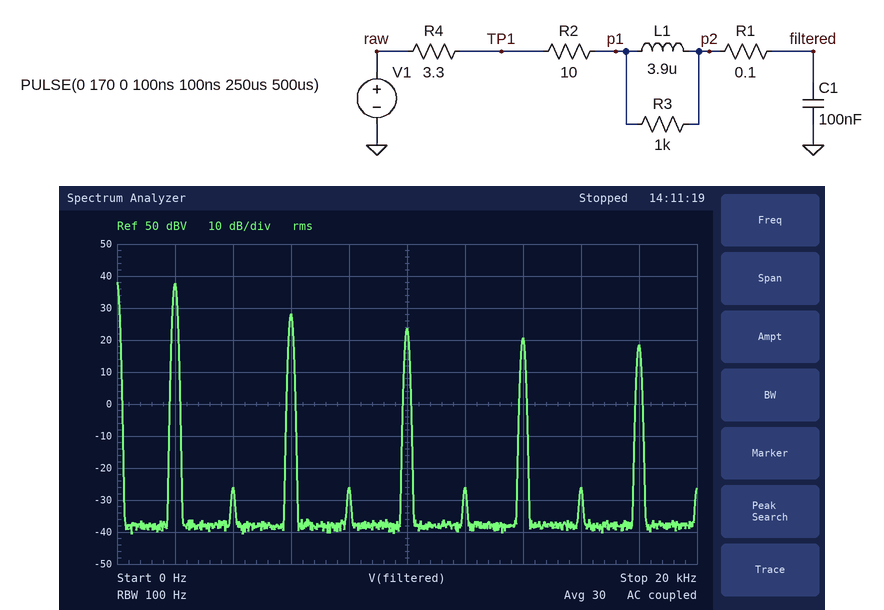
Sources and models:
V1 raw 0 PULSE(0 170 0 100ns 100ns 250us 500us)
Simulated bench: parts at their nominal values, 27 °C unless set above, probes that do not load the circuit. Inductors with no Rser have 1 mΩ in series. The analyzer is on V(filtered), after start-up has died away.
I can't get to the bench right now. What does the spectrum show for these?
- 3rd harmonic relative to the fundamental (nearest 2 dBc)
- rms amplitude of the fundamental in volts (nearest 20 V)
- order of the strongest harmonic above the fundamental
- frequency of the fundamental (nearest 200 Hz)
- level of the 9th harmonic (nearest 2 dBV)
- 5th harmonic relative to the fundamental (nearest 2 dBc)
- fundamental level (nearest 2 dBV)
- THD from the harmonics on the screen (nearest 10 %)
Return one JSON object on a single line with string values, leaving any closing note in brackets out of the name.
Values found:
{"3rd harmonic relative to the fundamental": "-10 dBc", "rms amplitude of the fundamental in volts": "80 V", "order of the strongest harmonic above the fundamental": "3", "frequency of the fundamental": "2.0 kHz", "level of the 9th harmonic": "18 dBV", "5th harmonic relative to the fundamental": "-14 dBc", "fundamental level": "38 dBV", "THD from the harmonics on the screen": "40 %"}
